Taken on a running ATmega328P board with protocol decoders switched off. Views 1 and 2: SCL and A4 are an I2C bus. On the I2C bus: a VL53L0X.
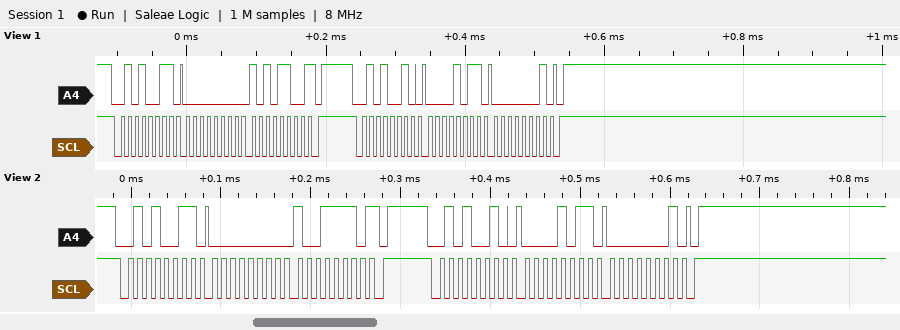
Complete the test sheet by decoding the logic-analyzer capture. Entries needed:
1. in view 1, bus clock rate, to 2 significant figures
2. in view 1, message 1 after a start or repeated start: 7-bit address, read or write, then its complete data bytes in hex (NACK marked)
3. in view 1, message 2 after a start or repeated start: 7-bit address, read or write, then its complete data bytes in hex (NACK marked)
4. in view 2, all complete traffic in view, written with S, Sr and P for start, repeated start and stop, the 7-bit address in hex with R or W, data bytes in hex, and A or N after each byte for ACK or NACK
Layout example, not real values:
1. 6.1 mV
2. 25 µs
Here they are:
1. 100 kHz
2. 0x29 read: 00 AC NACK
3. 0x29 write: 0B 01
4. S 29R A 00 A 9E N P S 29W A 0B A 01 A P
